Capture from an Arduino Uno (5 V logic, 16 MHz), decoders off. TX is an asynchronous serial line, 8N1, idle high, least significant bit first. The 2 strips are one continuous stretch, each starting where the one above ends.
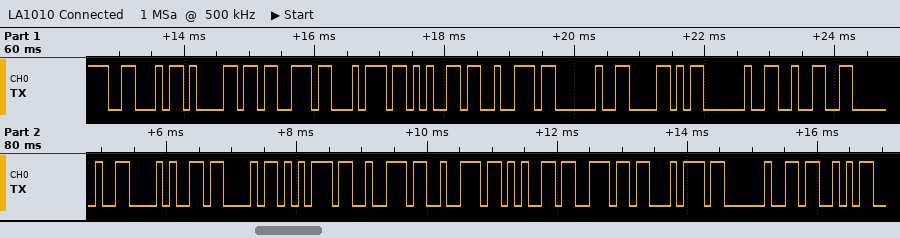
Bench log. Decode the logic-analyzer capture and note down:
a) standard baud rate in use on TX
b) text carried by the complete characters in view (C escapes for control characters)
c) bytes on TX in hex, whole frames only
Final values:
9600 baud
"Faster X 2 (Current S"
46 61 73 74 65 72 20 58 20 32 20 28 43 75 72 72 65 6E 74 20 53
